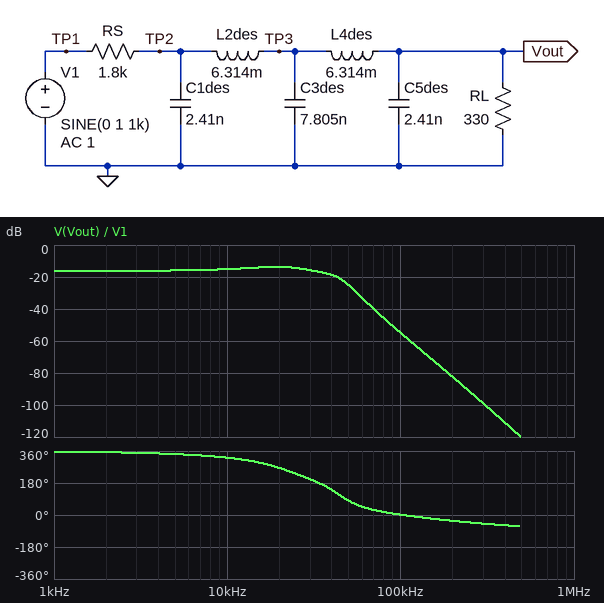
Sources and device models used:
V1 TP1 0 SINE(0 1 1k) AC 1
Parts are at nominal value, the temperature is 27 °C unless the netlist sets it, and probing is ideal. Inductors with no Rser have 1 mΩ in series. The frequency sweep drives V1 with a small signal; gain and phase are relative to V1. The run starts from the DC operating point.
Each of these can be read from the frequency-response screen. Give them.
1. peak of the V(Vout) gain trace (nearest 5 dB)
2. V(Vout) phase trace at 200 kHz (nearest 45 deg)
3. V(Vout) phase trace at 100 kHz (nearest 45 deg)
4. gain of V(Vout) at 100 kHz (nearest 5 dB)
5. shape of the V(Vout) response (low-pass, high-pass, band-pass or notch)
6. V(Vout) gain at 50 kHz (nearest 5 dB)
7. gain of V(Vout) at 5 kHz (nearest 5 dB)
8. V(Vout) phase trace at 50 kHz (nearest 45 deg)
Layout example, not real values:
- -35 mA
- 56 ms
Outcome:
- -15 dB
- -45 deg
- 0 deg
- -55 dB
- low-pass
- -25 dB
- -15 dB
- 90 deg
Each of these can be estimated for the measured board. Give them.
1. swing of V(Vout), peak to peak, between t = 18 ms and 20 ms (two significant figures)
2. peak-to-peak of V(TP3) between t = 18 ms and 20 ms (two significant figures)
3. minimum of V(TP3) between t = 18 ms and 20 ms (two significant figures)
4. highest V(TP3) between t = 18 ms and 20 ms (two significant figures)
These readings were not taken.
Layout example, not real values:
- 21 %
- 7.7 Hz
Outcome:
- 310 mV
- 310 mV
- -160 mV
- 160 mV
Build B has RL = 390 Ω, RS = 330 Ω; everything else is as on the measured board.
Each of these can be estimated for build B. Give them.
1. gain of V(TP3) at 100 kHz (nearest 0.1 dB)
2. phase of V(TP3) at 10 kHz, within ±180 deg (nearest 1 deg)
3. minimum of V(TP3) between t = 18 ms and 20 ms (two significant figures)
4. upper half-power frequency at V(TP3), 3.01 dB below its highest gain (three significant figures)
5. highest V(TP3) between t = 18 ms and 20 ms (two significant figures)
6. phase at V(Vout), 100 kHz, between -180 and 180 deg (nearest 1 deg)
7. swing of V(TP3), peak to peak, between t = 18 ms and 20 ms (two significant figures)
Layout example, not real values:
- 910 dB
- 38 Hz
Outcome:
- -25.5 dB
- -11 deg
- -540 mV
- 36.6 kHz
- 540 mV
- 42 deg
- 1.1 V
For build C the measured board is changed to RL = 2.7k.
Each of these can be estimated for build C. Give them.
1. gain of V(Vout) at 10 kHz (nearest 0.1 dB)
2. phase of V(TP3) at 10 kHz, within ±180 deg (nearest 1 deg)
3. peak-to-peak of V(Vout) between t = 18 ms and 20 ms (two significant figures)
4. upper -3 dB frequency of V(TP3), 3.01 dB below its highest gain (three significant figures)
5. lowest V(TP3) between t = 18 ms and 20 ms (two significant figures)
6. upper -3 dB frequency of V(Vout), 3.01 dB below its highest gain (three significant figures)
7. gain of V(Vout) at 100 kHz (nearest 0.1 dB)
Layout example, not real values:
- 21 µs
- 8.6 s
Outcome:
- -5.8 dB
- -44 deg
- 1.2 V
- 14.7 kHz
- -600 mV
- 49.4 kHz
- -46.9 dB
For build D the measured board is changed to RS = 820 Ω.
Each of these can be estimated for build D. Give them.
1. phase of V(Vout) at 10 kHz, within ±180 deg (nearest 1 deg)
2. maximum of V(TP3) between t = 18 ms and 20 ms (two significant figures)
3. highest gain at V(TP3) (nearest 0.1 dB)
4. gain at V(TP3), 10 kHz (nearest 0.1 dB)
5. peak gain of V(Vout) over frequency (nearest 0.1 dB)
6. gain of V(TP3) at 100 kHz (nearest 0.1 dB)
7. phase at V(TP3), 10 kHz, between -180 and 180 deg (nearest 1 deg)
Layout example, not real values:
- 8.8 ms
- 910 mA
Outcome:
- -49 deg
- 290 mV
- 0.8 dB
- -7.6 dB
- -10.7 dB
- -27.9 dB
- 3 deg
